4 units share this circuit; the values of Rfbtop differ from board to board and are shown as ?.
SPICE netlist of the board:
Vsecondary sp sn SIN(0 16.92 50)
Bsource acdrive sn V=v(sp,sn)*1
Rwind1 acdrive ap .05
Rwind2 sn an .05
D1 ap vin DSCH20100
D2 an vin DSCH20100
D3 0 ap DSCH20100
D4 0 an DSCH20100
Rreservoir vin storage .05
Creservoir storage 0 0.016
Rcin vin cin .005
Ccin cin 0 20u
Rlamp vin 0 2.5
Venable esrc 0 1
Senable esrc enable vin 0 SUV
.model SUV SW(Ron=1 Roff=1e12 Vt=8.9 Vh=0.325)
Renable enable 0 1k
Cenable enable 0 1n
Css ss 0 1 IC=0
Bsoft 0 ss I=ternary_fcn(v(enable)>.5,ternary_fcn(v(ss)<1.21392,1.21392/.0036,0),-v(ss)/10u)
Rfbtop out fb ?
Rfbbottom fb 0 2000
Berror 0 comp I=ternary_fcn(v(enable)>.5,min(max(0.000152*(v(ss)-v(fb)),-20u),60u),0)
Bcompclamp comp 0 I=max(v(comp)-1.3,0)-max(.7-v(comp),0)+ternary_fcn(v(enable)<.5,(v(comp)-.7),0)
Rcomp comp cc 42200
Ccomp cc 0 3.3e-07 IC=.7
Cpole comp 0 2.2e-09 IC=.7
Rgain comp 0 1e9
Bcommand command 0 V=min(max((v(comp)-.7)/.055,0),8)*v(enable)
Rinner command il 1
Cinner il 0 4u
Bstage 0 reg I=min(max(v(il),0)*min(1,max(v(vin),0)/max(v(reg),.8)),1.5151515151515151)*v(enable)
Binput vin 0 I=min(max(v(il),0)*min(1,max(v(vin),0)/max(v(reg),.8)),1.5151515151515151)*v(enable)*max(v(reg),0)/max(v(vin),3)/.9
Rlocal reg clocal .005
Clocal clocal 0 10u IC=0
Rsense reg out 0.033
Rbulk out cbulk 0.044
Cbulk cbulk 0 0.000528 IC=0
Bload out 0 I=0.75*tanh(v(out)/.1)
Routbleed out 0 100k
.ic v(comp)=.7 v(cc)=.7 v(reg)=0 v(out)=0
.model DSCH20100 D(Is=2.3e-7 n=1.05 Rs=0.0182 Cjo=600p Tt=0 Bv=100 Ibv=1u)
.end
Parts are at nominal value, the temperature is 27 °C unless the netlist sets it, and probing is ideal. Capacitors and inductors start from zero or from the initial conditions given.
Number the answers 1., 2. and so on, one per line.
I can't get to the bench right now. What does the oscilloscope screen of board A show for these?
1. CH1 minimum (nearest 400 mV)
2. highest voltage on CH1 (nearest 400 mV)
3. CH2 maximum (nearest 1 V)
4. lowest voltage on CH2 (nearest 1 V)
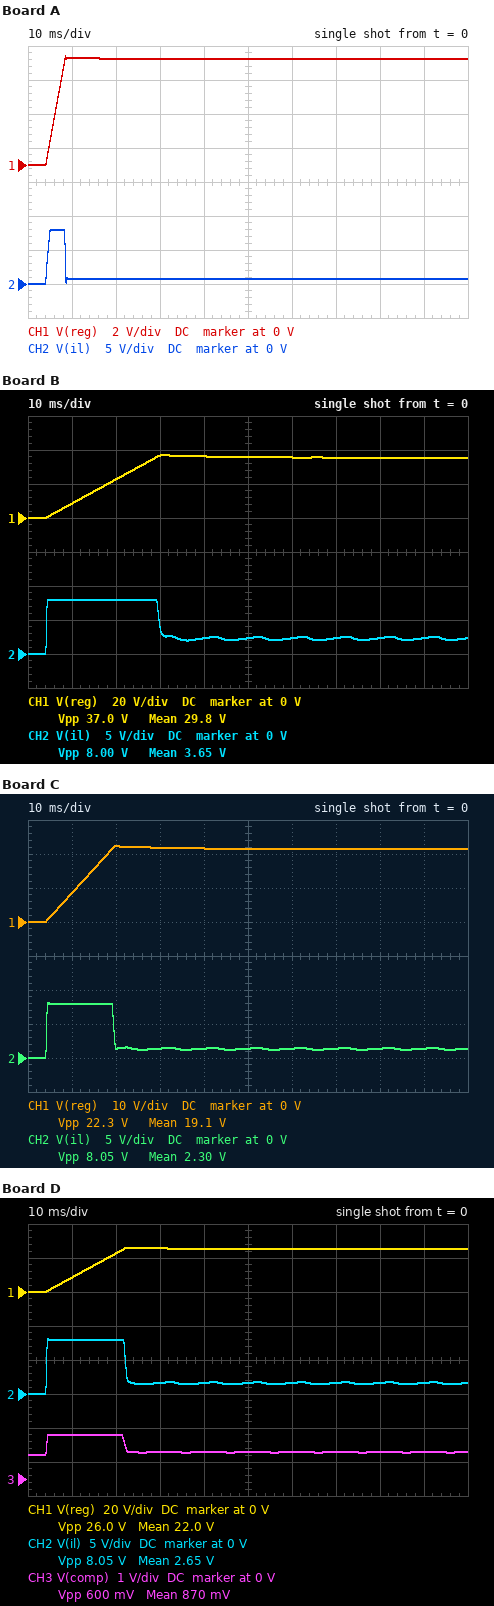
1. 0 V
2. 6.4 V
3. 8 V
4. 0 V
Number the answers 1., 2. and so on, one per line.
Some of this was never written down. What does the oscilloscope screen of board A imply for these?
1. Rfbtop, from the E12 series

1. 8.2 kΩ
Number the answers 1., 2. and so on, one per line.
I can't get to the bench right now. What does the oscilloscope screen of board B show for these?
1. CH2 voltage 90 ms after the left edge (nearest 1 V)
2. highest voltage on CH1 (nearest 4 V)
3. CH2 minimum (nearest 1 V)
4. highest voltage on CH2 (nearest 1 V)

1. 2 V
2. 36 V
3. 0 V
4. 8 V
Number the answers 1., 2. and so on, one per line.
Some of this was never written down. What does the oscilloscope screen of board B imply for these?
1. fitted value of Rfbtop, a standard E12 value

1. 56 kΩ
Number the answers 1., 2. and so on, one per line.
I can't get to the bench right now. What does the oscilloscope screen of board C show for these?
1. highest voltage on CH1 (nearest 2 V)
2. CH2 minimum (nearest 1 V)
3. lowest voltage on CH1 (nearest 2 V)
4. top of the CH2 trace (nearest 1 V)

1. 22 V
2. 0 V
3. 0 V
4. 8 V
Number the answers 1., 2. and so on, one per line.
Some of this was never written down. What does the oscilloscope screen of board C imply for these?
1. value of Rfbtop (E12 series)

1. 33 kΩ
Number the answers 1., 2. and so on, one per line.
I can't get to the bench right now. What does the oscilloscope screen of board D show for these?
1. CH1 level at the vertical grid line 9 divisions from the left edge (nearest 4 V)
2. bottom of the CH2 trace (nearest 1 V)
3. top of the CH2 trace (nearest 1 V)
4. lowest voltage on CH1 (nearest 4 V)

1. 24 V
2. 0 V
3. 8 V
4. 0 V
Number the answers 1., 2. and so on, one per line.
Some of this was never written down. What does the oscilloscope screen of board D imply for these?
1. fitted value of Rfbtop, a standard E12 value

1. 39 kΩ
